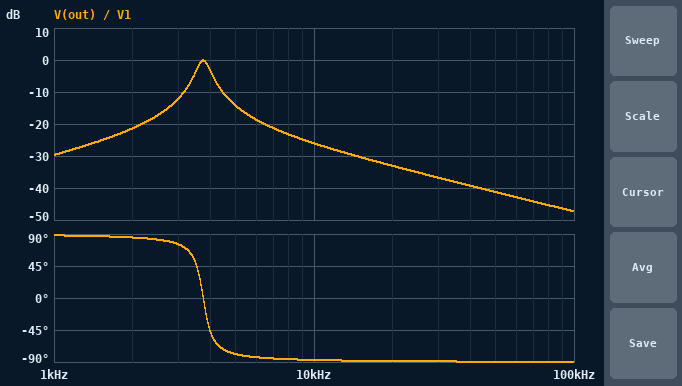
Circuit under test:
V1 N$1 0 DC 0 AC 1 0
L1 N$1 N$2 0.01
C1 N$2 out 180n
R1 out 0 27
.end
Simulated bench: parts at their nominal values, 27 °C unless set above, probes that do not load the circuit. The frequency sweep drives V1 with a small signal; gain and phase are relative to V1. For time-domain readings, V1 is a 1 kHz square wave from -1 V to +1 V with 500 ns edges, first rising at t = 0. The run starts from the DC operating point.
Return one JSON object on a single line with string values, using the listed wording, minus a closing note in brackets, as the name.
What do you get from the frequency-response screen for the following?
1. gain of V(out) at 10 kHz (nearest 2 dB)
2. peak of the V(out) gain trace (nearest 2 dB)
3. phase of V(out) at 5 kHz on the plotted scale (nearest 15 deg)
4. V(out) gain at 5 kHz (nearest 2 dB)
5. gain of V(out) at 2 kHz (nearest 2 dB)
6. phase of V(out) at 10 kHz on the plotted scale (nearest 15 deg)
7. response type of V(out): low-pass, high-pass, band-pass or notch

{"gain of V(out) at 10 kHz": "-26 dB", "peak of the V(out) gain trace": "0 dB", "phase of V(out) at 5 kHz on the plotted scale": "-75 deg", "V(out) gain at 5 kHz": "-14 dB", "gain of V(out) at 2 kHz": "-22 dB", "phase of V(out) at 10 kHz on the plotted scale": "-90 deg", "response type of V(out): low-pass, high-pass, band-pass or notch": "band-pass"}
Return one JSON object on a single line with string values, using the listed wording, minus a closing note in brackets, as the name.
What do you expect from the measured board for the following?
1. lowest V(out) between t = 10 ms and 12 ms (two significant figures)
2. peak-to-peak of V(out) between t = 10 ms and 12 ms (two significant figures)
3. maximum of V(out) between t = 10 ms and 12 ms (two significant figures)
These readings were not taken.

{"lowest V(out) between t = 10 ms and 12 ms": "-150 mV", "peak-to-peak of V(out) between t = 10 ms and 12 ms": "300 mV", "maximum of V(out) between t = 10 ms and 12 ms": "150 mV"}
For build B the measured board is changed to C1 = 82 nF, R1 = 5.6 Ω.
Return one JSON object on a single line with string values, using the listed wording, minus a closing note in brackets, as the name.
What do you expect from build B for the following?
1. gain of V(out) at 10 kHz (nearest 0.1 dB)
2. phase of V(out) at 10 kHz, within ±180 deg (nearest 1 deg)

{"gain of V(out) at 10 kHz": "-37.8 dB", "phase of V(out) at 10 kHz, within ±180 deg": "-89 deg"}
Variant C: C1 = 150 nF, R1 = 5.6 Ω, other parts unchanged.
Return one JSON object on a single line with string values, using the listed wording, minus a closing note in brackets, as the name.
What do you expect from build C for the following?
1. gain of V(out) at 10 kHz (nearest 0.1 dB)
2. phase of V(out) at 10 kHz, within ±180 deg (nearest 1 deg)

{"gain of V(out) at 10 kHz": "-39.4 dB", "phase of V(out) at 10 kHz, within ±180 deg": "-89 deg"}
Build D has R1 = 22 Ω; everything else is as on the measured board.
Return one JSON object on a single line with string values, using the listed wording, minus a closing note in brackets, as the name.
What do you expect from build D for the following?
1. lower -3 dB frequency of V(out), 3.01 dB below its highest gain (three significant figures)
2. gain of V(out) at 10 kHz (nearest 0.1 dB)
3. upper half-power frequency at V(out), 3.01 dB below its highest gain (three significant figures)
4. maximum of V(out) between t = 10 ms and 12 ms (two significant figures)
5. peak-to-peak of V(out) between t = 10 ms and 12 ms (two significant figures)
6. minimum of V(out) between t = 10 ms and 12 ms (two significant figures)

{"lower -3 dB frequency of V(out), 3.01 dB below its highest gain": "3.58 kHz", "gain of V(out) at 10 kHz": "-27.8 dB", "upper half-power frequency at V(out), 3.01 dB below its highest gain": "3.93 kHz", "maximum of V(out) between t = 10 ms and 12 ms": "120 mV", "peak-to-peak of V(out) between t = 10 ms and 12 ms": "240 mV", "minimum of V(out) between t = 10 ms and 12 ms": "-120 mV"}
